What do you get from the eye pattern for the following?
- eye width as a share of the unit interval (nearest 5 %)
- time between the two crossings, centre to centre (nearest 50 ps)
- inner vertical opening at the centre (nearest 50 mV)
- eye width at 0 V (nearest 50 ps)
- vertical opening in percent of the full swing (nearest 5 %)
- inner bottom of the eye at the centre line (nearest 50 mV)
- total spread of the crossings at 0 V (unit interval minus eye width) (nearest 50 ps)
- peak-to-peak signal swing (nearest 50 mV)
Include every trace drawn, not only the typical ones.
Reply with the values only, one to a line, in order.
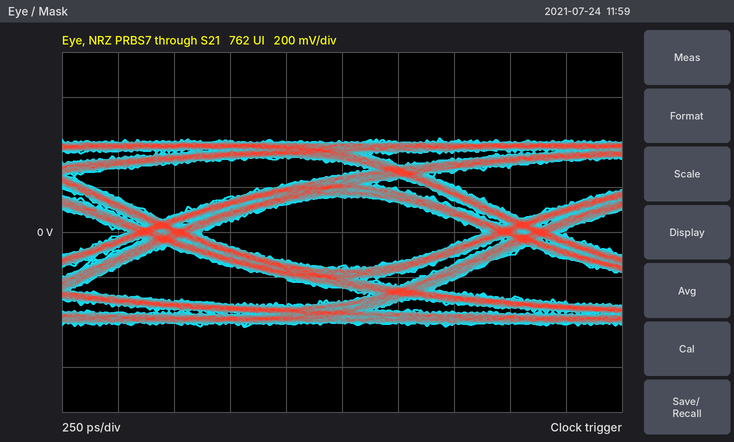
80 %
1.60 ns
300 mV
1.25 ns
35 %
-150 mV
350 ps
850 mV
